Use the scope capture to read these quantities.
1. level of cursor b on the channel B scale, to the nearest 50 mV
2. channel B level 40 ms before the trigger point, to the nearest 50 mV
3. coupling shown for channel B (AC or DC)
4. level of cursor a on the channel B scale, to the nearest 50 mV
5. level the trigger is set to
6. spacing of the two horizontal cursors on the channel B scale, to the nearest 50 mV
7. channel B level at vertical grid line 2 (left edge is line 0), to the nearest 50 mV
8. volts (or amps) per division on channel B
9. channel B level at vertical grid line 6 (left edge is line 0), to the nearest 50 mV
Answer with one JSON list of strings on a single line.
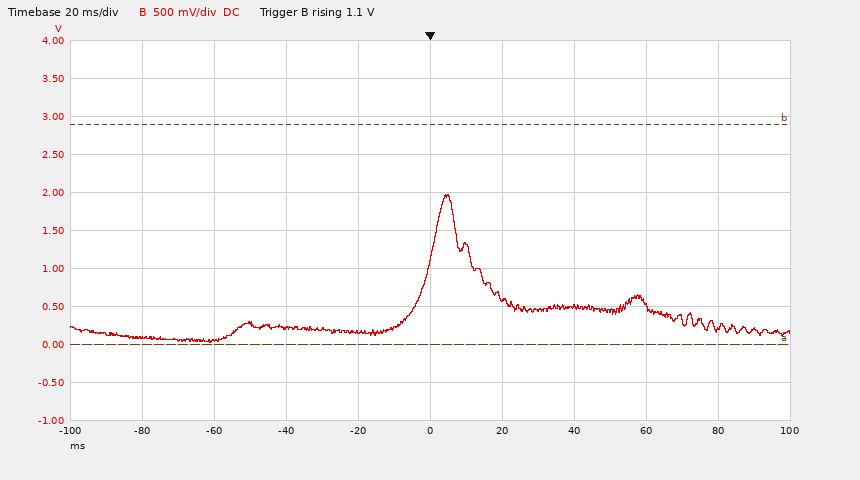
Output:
["2.90 V", "200 mV", "DC", "0 mV", "1.1 V", "2.90 V", "50 mV", "500 mV", "600 mV"]
